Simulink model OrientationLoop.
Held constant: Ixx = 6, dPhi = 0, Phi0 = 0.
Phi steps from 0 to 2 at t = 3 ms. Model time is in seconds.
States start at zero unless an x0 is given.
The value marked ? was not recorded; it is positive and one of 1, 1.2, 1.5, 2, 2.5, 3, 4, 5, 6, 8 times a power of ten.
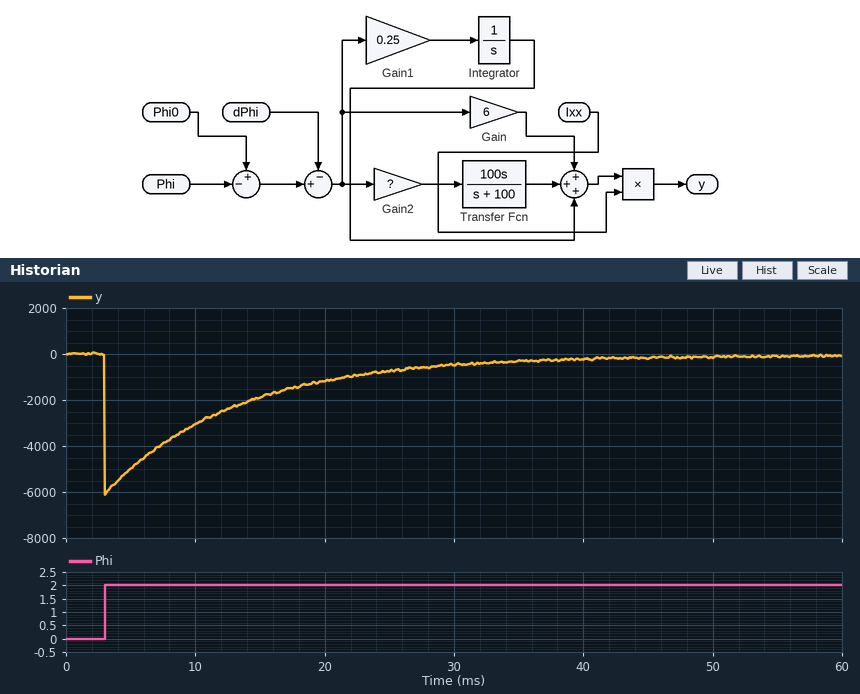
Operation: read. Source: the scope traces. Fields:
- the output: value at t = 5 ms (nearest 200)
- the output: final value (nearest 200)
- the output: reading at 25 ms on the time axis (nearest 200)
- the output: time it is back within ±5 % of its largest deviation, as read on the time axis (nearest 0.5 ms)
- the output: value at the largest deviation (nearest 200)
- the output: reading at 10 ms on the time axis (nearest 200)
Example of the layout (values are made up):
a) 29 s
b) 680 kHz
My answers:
a) -5000
b) 0
c) -800
d) 33.0 ms
e) -6000
f) -3000
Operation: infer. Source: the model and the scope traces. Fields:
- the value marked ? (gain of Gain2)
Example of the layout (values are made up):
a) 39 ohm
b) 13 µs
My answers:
a) 5
